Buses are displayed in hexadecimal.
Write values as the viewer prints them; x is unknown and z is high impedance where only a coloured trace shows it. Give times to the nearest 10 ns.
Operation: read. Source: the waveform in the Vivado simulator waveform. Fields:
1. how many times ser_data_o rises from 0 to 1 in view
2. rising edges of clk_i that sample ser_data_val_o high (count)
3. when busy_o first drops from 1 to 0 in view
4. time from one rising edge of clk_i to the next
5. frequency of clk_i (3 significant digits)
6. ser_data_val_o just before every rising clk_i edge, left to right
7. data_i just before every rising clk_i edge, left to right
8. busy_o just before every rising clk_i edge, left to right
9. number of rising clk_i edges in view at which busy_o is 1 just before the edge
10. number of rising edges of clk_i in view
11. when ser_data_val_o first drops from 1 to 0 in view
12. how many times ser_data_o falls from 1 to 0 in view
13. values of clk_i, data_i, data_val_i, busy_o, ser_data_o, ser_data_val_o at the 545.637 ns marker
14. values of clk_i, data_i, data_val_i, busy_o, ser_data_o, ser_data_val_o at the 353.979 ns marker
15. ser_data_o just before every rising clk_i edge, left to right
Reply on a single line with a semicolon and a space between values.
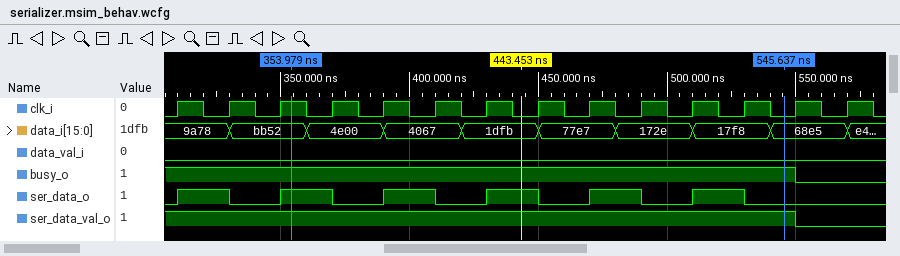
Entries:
6; 13; 550 ns; 20 ns; 50.0 MHz; 1 1 1 1 1 1 1 1 1 1 1 1 1 0; 9a78, 9a78, bb52, 4e00, 4e00, 4067, 1dfb, 1dfb, 77e7, 172e, 172e, 17f8, 68e5, 68e5; 1 1 1 1 1 1 1 1 1 1 1 1 1 0; 13; 14; 550 ns; 6; clk_i=0, data_i=68e5, data_val_i=0, busy_o=1, ser_data_o=0, ser_data_val_o=1; clk_i=1, data_i=bb52, data_val_i=0, busy_o=1, ser_data_o=1, ser_data_val_o=1; 0 1 0 1 0 1 0 1 0 1 0 1 0 0
